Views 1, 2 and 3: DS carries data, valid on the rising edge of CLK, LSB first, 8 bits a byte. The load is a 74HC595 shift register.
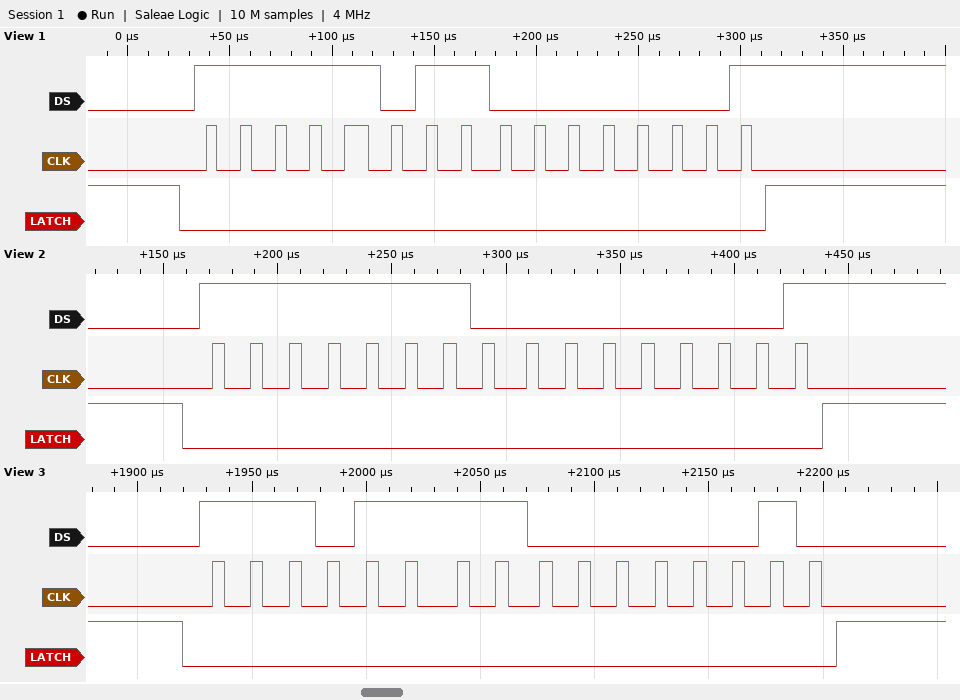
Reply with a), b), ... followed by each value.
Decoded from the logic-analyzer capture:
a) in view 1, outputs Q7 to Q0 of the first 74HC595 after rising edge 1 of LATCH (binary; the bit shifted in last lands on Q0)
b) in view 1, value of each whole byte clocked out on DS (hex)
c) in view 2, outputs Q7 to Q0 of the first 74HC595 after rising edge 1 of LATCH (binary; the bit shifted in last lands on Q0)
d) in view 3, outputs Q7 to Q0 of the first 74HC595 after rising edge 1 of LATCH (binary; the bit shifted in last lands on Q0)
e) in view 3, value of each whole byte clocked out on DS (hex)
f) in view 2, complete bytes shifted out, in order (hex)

a) 00000001
b) DF 80
c) 00000001
d) 00000010
e) F7 40
f) 7F 80
